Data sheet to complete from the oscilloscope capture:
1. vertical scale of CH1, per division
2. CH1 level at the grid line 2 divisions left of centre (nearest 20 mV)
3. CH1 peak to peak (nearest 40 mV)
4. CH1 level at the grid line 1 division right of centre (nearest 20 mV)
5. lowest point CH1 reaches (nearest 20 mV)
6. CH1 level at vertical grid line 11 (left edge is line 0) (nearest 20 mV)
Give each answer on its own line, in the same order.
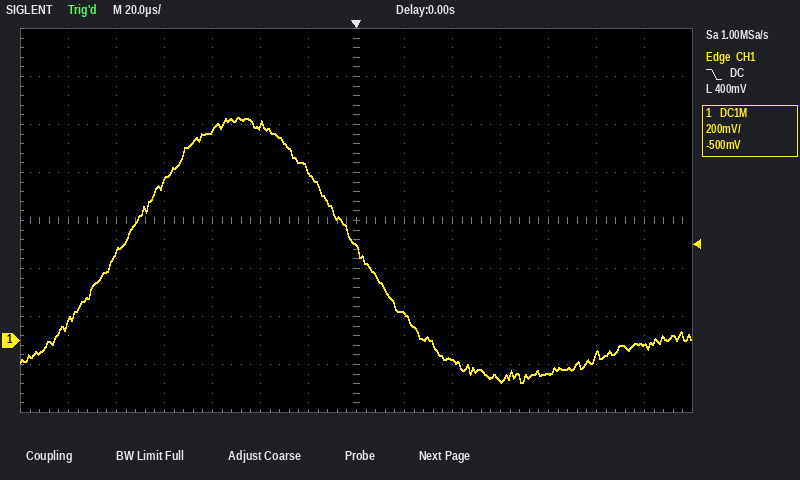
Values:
200 mV
900 mV
1.12 V
120 mV
-180 mV
-140 mV
